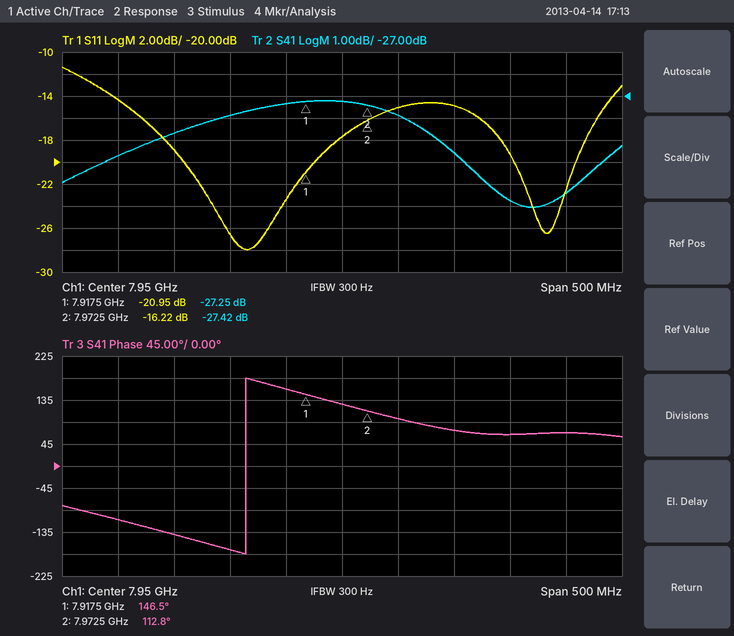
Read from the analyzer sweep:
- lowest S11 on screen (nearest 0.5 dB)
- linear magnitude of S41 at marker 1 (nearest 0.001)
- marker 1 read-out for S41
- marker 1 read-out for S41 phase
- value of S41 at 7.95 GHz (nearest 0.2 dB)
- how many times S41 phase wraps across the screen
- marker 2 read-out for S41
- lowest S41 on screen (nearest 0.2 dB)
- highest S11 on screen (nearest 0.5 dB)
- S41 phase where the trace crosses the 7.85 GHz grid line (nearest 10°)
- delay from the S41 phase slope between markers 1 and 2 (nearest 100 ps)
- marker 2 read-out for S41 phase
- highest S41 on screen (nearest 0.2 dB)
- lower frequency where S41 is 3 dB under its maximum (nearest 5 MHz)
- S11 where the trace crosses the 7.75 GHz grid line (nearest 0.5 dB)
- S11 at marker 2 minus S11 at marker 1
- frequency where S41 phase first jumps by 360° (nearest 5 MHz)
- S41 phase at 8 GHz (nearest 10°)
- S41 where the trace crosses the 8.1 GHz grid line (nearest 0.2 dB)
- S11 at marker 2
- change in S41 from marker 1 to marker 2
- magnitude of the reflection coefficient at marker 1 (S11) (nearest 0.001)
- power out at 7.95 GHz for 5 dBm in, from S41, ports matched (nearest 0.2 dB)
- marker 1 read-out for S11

-28.0 dB
0.043
-27.25 dB
146.5°
-27.2 dB
1
-27.42 dB
-32.0 dB
-11.5 dB
-170°
1.7 ns
112.8°
-27.2 dB
7.730 GHz
-14.5 dB
4.73 dB
7.865 GHz
100°
-31.8 dB
-16.22 dB
-0.17 dB
0.090
-22.2 dBm
-20.95 dB
